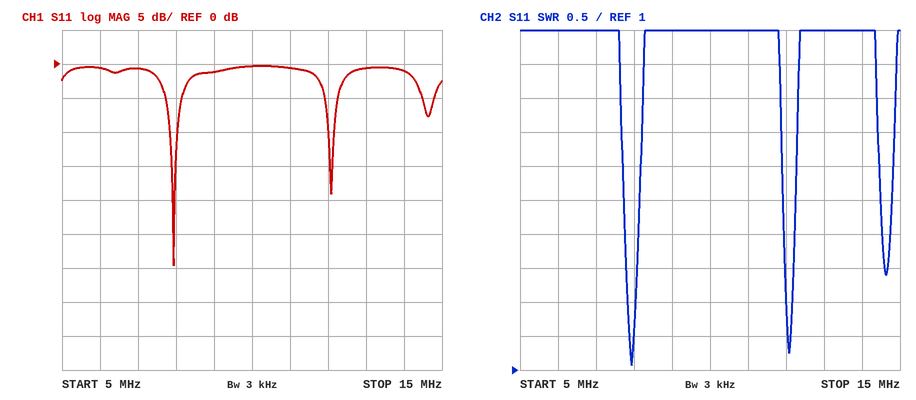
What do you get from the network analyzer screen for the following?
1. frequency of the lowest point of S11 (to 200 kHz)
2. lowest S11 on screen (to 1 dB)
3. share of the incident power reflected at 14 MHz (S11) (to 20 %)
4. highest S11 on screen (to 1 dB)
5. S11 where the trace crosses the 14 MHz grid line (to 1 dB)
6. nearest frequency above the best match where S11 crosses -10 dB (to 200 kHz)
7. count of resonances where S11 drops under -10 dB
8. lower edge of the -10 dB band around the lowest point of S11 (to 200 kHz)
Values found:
8.0 MHz
-30 dB
80 %
0 dB
-1 dB
8.0 MHz
2
7.8 MHz
